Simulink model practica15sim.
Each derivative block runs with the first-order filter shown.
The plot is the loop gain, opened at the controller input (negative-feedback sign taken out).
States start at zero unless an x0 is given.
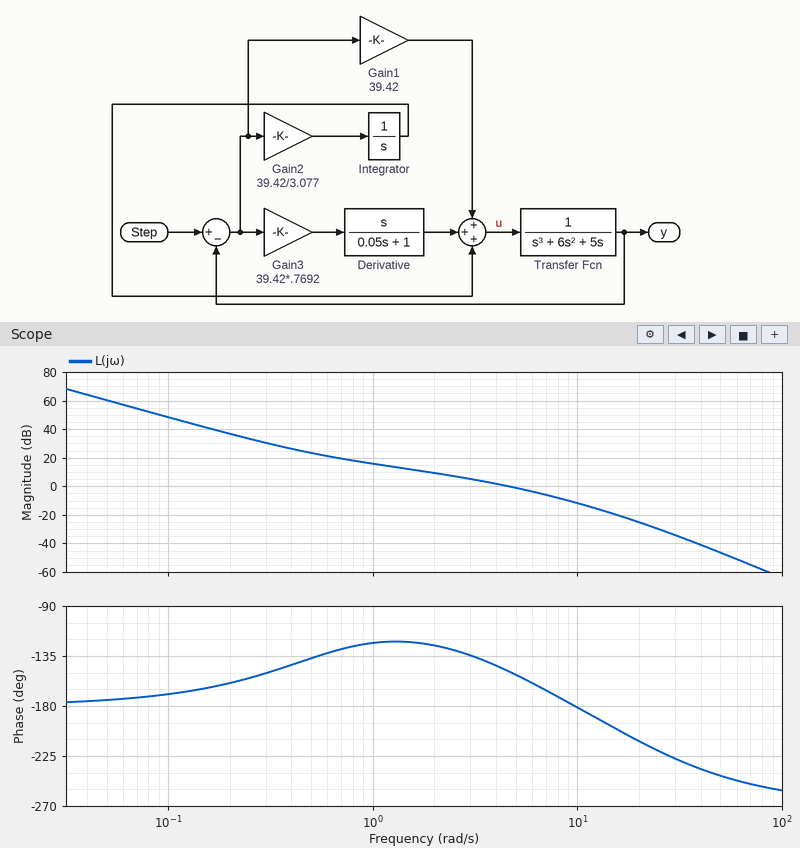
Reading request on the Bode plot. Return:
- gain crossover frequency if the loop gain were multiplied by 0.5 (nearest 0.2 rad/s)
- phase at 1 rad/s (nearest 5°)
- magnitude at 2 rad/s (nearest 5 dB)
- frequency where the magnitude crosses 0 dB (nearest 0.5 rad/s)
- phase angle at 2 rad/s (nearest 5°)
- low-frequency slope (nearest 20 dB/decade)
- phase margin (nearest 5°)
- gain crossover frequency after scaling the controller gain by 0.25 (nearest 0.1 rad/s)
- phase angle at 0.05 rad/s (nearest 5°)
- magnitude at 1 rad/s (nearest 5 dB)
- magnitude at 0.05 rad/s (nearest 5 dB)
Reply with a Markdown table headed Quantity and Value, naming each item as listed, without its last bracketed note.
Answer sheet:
| Quantity | Value |
|---|---|
| gain crossover frequency if the loop gain were multiplied by 0.5 | 2.8 rad/s |
| phase at 1 rad/s | -125° |
| magnitude at 2 rad/s | 10 dB |
| frequency where the magnitude crosses 0 dB | 4.5 rad/s |
| phase angle at 2 rad/s | -125° |
| low-frequency slope | -40 dB/decade |
| phase margin | 30° |
| gain crossover frequency after scaling the controller gain by 0.25 | 1.5 rad/s |
| phase angle at 0.05 rad/s | -175° |
| magnitude at 1 rad/s | 15 dB |
| magnitude at 0.05 rad/s | 60 dB |
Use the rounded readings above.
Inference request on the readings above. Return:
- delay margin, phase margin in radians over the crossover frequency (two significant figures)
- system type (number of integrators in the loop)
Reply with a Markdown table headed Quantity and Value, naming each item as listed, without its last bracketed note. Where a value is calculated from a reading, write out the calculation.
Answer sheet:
| Quantity | Value |
|---|---|
| delay margin, phase margin in radians over the crossover frequency | 30 × π / 180 / 4.5 = 0.12 s |
| system type | 2 |
